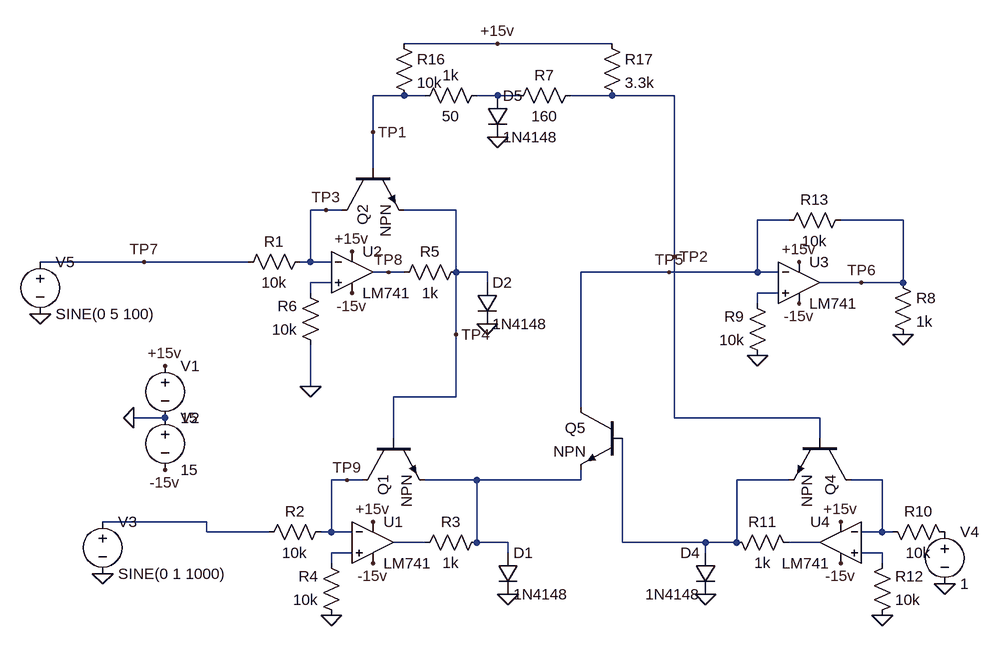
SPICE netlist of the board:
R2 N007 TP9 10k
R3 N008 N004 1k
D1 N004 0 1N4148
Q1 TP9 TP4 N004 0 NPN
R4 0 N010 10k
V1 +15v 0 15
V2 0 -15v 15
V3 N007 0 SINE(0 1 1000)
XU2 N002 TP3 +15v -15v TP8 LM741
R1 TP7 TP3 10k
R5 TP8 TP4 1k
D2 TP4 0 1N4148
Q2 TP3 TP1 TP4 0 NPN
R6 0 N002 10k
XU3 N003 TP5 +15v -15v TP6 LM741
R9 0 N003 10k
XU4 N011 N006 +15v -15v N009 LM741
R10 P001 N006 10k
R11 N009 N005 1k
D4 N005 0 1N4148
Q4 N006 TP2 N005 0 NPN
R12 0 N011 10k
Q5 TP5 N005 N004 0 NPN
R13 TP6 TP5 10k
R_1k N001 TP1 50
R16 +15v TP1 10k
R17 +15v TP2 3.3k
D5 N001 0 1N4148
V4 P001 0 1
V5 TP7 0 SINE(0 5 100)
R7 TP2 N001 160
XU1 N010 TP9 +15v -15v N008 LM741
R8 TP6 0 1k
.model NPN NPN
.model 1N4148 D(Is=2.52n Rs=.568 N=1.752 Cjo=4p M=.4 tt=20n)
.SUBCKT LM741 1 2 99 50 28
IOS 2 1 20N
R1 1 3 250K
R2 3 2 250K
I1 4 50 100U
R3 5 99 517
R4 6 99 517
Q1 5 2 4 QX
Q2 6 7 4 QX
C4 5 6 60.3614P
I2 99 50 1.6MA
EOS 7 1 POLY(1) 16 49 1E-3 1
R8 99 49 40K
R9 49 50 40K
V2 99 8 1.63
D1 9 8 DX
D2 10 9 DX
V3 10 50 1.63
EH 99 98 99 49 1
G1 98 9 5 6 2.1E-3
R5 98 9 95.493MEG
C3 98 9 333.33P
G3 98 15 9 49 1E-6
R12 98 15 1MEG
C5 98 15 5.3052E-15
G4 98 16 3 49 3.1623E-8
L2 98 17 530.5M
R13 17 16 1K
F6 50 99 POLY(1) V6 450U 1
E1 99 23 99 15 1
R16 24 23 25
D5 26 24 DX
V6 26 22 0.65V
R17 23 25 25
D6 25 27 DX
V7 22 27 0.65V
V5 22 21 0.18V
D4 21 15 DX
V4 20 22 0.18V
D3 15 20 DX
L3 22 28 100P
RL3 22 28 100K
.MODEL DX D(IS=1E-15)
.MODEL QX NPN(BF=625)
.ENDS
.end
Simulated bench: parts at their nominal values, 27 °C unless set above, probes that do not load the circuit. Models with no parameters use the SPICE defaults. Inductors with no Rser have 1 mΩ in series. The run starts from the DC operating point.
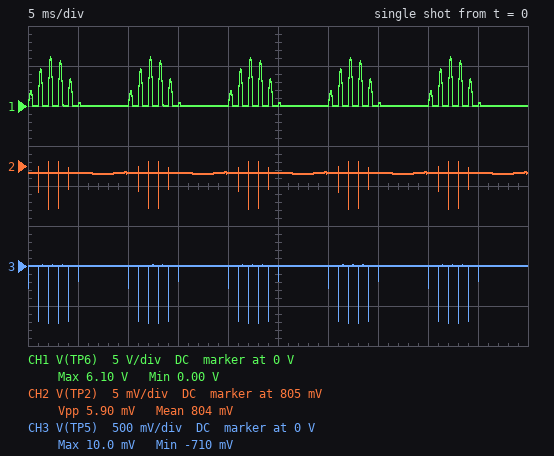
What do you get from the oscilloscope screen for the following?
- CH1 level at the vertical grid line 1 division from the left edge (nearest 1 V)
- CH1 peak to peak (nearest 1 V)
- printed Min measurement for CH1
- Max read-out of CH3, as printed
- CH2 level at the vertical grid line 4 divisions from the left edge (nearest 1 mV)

0 V
6 V
0.00 V
10.0 mV
804 mV
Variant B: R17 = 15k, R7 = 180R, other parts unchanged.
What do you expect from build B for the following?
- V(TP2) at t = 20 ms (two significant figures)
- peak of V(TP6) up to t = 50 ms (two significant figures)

740 mV
6.8 V
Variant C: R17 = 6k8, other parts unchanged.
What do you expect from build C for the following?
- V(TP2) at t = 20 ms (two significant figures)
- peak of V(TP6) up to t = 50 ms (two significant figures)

780 mV
6.5 V
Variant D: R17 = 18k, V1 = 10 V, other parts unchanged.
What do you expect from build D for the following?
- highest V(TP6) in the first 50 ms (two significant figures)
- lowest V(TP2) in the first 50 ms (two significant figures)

8.7 V
670 mV
